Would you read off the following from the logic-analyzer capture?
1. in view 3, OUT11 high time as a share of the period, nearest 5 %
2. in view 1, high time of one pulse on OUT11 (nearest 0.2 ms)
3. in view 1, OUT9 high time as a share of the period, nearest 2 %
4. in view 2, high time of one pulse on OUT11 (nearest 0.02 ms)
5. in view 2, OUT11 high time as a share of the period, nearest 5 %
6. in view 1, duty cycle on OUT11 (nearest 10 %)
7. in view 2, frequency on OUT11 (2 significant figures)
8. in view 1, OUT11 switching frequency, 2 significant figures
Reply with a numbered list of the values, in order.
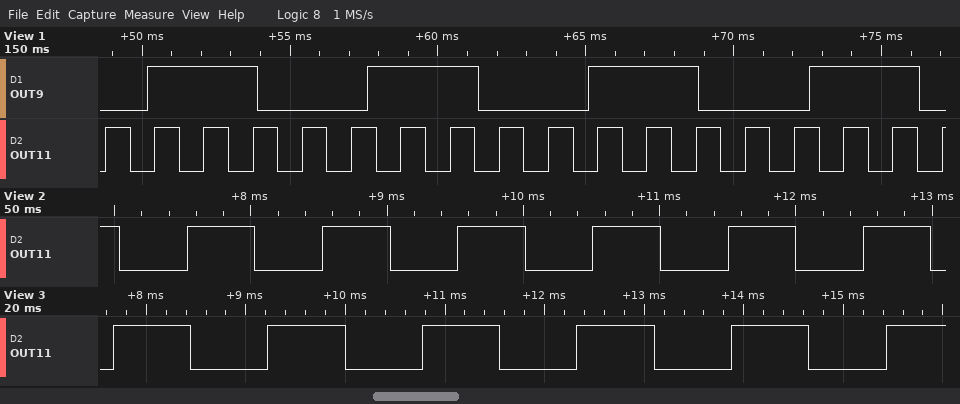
1. 50 %
2. 0.8 ms
3. 50 %
4. 0.50 ms
5. 50 %
6. 50 %
7. 1.0 kHz
8. 600 Hz
